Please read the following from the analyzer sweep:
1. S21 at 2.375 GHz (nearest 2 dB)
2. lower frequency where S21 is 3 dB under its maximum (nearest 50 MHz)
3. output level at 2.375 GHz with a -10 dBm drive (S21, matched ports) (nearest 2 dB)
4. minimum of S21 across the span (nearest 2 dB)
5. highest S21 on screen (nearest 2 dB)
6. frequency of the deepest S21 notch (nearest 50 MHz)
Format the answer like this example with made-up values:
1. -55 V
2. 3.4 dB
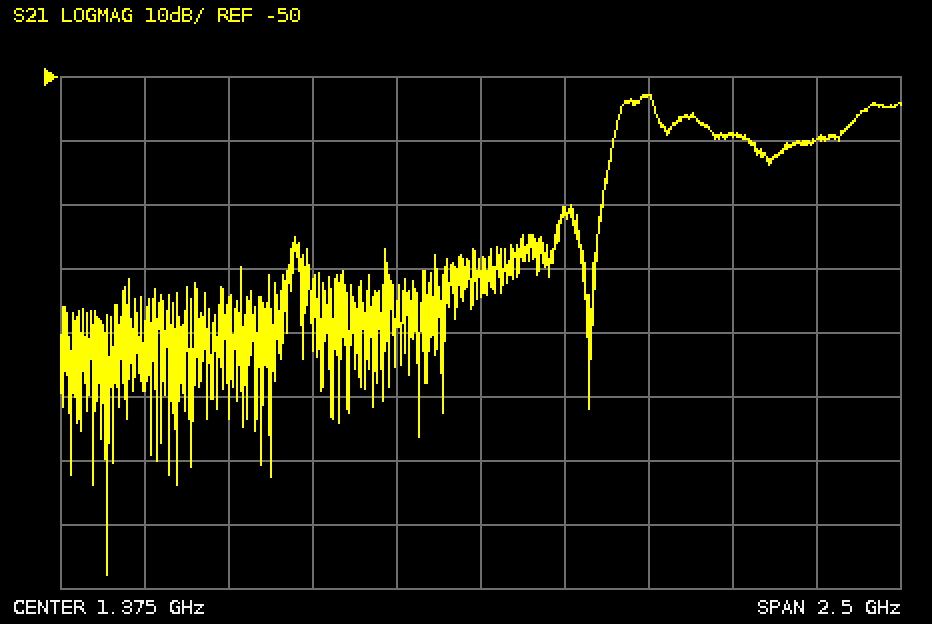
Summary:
1. -60 dB
2. 1.80 GHz
3. -70 dBm
4. -128 dB
5. -52 dB
6. 250 MHz
